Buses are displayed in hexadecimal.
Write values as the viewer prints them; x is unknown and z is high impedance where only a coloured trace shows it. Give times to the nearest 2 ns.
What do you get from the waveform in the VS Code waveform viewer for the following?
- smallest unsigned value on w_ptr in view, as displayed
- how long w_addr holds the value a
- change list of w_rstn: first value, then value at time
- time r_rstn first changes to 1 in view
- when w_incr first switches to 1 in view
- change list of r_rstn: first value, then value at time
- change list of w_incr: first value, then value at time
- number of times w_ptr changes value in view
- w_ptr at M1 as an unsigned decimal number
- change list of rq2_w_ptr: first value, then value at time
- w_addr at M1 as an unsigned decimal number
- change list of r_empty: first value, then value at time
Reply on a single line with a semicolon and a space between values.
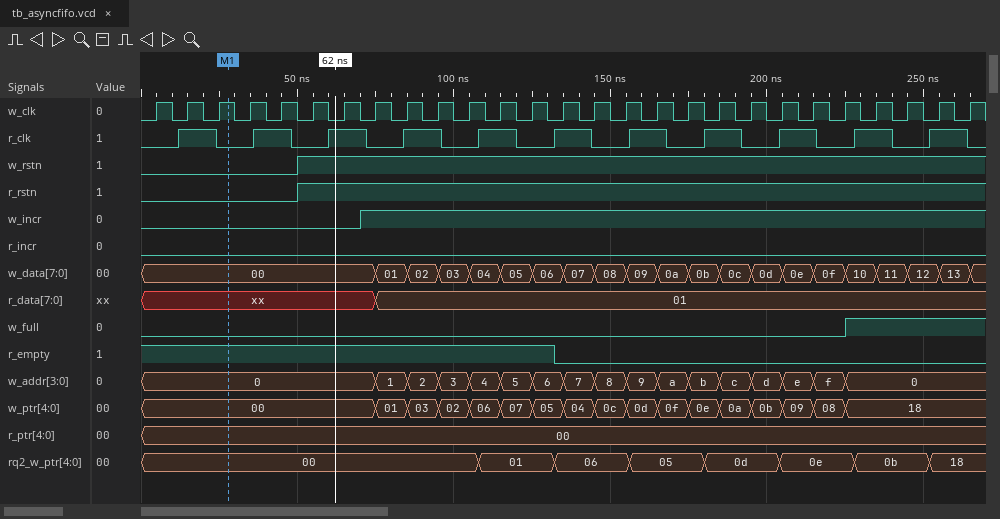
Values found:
00; 10 ns; 0, 1 at 50 ns; 50 ns; 70 ns; 0, 1 at 50 ns; 0, 1 at 70 ns; 16; 0; 00, 01 at 108 ns, 06 at 132 ns, 05 at 156 ns, 0d at 180 ns, 0e at 204 ns, 0b at 228 ns, 18 at 252 ns; 0; 1, 0 at 132 ns
